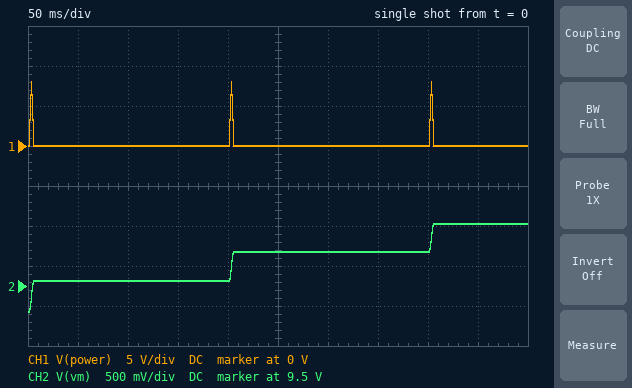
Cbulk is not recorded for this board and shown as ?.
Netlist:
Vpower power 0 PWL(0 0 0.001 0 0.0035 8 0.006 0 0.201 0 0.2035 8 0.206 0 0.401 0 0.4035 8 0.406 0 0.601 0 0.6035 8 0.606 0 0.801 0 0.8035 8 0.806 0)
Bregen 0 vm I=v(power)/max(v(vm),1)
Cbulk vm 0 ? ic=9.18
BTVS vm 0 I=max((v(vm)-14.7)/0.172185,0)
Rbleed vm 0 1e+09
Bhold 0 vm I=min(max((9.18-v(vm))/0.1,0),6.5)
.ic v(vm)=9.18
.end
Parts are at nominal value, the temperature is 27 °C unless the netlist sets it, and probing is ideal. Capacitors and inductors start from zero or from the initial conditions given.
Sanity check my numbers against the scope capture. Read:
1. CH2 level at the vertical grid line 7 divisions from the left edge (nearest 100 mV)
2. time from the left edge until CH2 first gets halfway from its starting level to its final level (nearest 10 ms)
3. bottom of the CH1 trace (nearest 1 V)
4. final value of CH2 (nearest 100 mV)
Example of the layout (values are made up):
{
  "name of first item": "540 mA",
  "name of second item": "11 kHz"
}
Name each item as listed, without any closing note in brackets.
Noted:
{
  "CH2 level at the vertical grid line 7 divisions from the left edge": "9.9 V",
  "time from the left edge until CH2 first gets halfway from its starting level to its final level": "200 ms",
  "bottom of the CH1 trace": "0 V",
  "final value of CH2": "10.3 V"
}
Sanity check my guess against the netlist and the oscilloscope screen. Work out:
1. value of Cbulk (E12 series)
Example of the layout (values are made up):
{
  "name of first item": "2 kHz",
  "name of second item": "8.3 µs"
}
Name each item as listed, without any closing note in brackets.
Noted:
{
  "value of Cbulk": "5.6 mF"
}
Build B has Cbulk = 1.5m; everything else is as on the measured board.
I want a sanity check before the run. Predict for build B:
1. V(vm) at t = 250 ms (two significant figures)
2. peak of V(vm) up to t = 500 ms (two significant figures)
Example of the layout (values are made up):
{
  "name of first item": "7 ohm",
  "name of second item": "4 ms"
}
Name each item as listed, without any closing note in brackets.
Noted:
{
  "V(vm) at t = 250 ms": "12 V",
  "peak of V(vm) up to t = 500 ms": "13 V"
}
